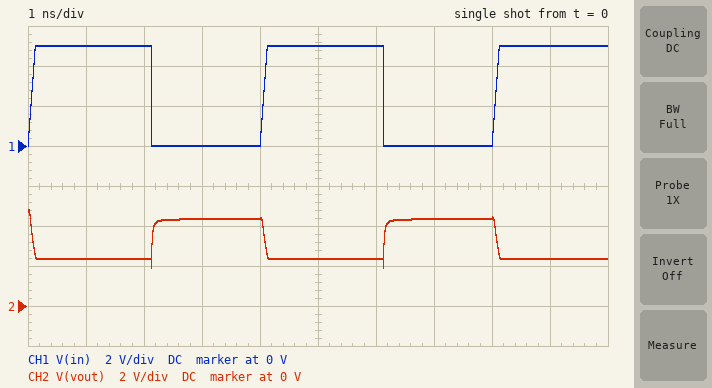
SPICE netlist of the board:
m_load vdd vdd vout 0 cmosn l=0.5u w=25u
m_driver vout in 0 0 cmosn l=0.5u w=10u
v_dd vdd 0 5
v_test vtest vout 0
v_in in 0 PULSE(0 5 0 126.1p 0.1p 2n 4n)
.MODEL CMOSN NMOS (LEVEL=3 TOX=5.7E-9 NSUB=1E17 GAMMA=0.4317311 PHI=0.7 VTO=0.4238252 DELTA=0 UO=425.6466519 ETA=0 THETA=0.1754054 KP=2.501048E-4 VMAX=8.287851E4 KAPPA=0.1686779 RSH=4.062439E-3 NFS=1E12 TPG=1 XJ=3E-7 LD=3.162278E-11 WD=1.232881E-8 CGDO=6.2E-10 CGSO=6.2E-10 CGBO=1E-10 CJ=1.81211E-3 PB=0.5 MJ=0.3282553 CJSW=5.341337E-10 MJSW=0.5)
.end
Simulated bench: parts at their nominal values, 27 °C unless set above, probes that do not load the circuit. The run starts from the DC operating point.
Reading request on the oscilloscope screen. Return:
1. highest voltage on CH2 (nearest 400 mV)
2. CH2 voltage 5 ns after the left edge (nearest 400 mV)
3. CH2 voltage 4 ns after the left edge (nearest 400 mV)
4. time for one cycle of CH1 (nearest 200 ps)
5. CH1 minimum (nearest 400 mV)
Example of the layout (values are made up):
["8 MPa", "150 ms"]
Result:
["4.8 V", "2.4 V", "4.4 V", "4.0 ns", "0 V"]
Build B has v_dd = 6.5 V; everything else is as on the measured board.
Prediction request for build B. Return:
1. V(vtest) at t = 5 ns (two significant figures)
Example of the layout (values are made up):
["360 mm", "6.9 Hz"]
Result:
["3.7 V"]
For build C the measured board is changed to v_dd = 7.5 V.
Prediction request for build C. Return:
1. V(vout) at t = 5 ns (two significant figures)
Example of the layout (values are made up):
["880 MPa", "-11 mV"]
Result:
["4.6 V"]
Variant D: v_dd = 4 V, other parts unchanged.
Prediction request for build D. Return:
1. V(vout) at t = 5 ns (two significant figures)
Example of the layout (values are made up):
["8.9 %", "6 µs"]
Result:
["1.5 V"]
